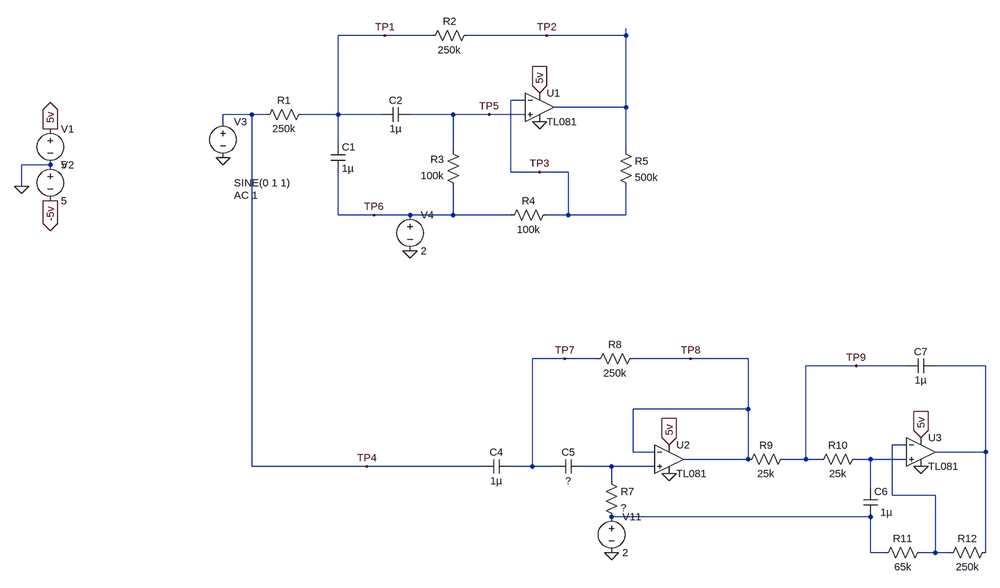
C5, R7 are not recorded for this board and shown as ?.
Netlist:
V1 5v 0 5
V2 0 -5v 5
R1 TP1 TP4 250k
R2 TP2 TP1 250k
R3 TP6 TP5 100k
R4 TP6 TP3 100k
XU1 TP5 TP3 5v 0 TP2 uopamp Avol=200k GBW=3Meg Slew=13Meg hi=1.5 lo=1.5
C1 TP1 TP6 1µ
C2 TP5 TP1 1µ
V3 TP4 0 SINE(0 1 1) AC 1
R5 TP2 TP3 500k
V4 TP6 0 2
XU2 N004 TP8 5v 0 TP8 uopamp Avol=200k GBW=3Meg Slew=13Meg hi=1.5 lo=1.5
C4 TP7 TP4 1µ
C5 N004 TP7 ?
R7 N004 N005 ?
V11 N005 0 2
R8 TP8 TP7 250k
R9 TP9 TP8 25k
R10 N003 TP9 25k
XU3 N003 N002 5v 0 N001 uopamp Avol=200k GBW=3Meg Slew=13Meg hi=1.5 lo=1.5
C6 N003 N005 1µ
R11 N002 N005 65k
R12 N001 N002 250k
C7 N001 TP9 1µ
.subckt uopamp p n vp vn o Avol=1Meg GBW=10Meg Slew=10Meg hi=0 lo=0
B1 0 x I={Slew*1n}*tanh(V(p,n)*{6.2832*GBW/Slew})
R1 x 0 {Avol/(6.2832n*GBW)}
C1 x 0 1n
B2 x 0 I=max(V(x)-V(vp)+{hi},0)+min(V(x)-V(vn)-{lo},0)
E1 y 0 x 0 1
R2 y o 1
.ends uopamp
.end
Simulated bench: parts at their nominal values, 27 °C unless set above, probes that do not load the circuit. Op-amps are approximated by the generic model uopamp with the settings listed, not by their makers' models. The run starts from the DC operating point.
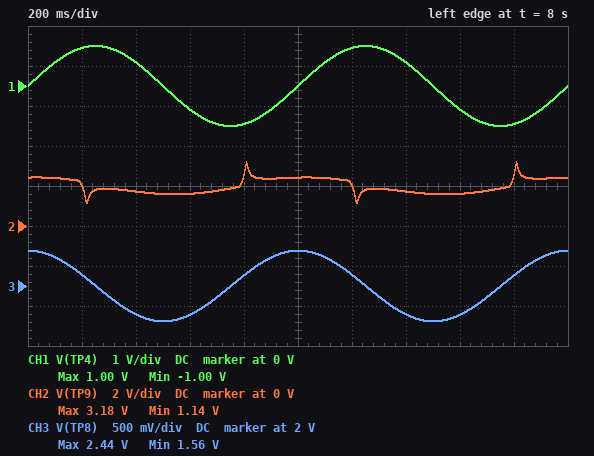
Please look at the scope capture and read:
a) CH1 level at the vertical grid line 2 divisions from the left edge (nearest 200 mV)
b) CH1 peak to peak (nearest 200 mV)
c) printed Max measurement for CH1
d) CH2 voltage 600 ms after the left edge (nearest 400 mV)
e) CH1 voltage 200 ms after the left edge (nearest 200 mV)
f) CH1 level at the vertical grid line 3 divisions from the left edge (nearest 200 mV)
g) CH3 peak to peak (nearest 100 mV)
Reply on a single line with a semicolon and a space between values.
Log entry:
600 mV; 2.0 V; 1.00 V; 1.6 V; 1.0 V; -600 mV; 900 mV
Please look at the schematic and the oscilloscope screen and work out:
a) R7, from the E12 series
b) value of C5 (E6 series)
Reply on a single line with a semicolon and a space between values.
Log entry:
220 kΩ; 470 nF
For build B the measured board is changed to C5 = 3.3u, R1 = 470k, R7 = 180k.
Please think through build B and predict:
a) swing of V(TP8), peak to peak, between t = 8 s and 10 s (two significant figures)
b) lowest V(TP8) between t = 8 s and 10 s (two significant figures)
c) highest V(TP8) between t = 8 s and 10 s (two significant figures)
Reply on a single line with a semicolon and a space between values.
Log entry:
1.2 V; 1.5 V; 2.7 V
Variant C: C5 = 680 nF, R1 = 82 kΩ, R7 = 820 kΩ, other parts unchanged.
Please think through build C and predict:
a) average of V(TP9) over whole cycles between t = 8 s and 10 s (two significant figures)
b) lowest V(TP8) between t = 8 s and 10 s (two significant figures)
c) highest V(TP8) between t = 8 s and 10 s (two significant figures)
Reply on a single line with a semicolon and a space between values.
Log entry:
2.1 V; 1.5 V; 3.0 V
